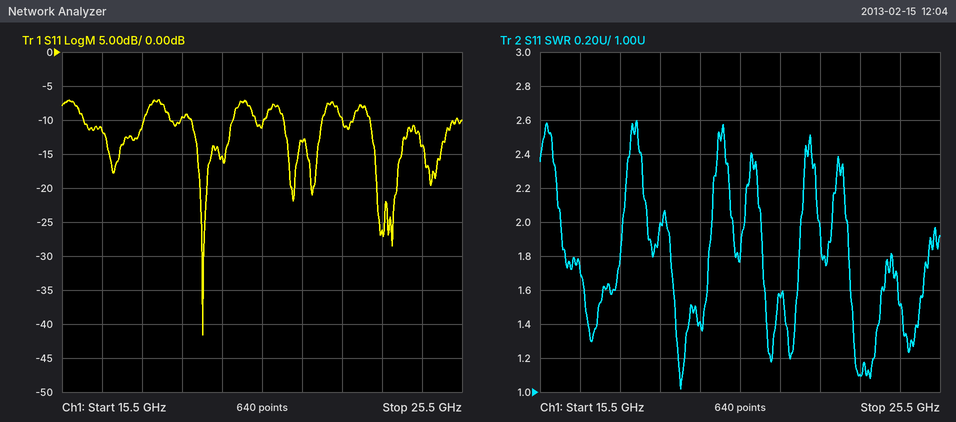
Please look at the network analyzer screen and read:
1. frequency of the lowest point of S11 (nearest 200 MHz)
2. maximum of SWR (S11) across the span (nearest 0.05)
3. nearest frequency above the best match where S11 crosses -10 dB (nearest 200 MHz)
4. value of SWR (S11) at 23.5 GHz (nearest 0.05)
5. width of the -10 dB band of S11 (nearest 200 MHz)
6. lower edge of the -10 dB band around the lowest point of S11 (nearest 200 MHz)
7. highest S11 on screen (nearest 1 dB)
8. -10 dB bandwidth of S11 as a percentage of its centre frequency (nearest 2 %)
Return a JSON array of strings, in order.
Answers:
["19.0 GHz", "2.60", "19.8 GHz", "1.10", "1.0 GHz", "18.8 GHz", "-7 dB", "6 %"]
